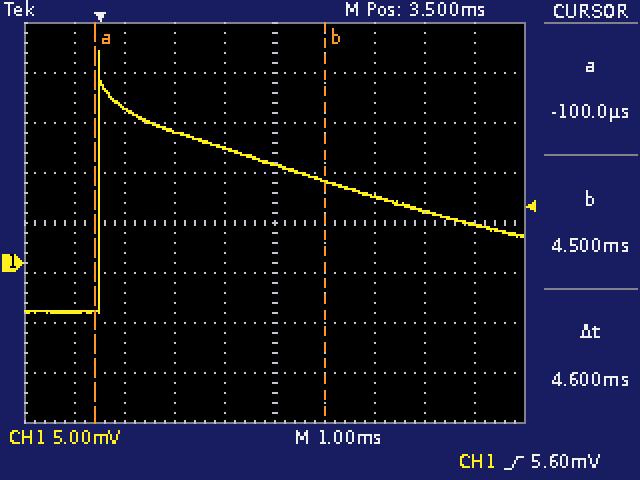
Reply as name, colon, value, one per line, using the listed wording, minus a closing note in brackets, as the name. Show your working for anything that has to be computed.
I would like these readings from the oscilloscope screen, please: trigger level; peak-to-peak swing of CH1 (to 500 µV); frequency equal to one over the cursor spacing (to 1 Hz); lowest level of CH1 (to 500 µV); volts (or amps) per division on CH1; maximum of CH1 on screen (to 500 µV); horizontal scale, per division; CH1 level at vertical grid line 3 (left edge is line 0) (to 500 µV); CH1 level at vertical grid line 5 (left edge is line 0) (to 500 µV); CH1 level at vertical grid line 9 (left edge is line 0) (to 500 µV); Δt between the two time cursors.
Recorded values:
trigger level: 5.60 mV
peak-to-peak swing of CH1: 21.0 mV − (-5.0 mV) = 26.0 mV
frequency equal to one over the cursor spacing: 1 / 4.6 ms ≈ 217 Hz
lowest level of CH1: -5.0 mV
volts (or amps) per division on CH1: 5 mV
maximum of CH1 on screen: 21.0 mV
horizontal scale, per division: 1 ms
CH1 level at vertical grid line 3 (left edge is line 0): 13.0 mV
CH1 level at vertical grid line 5 (left edge is line 0): 10.0 mV
CH1 level at vertical grid line 9 (left edge is line 0): 4.0 mV
Δt between the two time cursors: 4.6 ms
